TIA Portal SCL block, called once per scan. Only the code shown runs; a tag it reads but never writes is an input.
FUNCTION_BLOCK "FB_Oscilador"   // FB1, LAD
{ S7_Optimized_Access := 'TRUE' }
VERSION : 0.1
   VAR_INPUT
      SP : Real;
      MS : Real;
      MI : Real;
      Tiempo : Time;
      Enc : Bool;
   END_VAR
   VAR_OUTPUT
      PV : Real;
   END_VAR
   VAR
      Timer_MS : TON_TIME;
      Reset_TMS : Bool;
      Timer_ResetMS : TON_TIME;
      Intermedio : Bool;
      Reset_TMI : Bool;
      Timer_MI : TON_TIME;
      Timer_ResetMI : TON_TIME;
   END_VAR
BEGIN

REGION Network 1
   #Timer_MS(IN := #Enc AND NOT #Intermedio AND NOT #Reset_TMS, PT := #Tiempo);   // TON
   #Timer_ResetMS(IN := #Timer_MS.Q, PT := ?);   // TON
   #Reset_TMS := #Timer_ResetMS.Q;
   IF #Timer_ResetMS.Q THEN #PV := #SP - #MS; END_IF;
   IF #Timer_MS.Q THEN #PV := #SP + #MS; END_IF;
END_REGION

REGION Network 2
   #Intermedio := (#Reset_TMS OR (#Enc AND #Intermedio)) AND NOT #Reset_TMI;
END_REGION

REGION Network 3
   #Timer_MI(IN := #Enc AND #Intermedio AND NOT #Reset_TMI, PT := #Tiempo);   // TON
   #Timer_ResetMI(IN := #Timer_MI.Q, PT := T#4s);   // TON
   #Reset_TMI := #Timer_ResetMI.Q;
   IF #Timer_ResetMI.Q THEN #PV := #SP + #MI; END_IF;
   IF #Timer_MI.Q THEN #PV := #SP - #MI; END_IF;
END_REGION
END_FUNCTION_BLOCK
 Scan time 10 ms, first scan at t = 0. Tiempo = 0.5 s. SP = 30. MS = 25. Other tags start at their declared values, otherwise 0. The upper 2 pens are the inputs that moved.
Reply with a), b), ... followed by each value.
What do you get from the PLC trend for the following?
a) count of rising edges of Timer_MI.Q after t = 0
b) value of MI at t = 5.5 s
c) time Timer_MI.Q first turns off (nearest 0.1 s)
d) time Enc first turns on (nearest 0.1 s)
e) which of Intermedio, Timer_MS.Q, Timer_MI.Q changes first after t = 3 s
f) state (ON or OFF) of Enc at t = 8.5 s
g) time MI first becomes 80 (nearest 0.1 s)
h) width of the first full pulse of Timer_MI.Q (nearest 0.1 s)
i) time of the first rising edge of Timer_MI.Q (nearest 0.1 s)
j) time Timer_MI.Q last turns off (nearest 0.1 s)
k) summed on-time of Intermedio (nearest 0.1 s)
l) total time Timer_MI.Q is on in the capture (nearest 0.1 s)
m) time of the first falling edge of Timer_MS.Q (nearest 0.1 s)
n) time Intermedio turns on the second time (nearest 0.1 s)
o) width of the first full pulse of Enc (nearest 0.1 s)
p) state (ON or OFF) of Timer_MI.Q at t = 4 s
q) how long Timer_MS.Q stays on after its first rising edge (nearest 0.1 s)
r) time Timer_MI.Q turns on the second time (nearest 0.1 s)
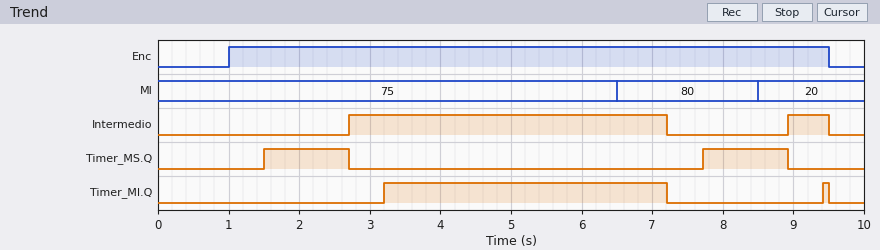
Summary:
a) 2
b) 75
c) 7.2 s
d) 1.0 s
e) Timer_MI.Q
f) ON
g) 6.5 s
h) 4.0 s
i) 3.2 s
j) 9.5 s
k) 5.1 s
l) 4.1 s
m) 2.7 s
n) 8.9 s
o) 8.5 s
p) ON
q) 1.2 s
r) 9.4 s
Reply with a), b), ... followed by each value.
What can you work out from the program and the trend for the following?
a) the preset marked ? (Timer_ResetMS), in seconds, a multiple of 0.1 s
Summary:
a) 1.2 s
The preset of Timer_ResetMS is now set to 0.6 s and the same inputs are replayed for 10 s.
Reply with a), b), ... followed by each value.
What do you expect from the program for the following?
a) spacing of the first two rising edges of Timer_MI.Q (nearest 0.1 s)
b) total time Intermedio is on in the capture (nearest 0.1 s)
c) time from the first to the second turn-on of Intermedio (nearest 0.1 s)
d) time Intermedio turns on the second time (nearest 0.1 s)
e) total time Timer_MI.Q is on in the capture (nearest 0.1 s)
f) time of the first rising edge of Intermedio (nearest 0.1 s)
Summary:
a) 5.6 s
b) 6.3 s
c) 5.6 s
d) 7.7 s
e) 5.3 s
f) 2.1 s
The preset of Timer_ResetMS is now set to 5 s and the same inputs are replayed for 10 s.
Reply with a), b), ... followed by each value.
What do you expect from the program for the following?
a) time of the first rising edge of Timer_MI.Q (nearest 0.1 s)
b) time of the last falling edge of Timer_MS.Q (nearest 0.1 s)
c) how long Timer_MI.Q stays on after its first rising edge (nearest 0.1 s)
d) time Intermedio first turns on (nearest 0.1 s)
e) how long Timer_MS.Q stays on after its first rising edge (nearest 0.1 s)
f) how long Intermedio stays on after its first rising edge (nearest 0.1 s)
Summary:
a) 7.0 s
b) 6.5 s
c) 2.5 s
d) 6.5 s
e) 5.0 s
f) 3.0 s
